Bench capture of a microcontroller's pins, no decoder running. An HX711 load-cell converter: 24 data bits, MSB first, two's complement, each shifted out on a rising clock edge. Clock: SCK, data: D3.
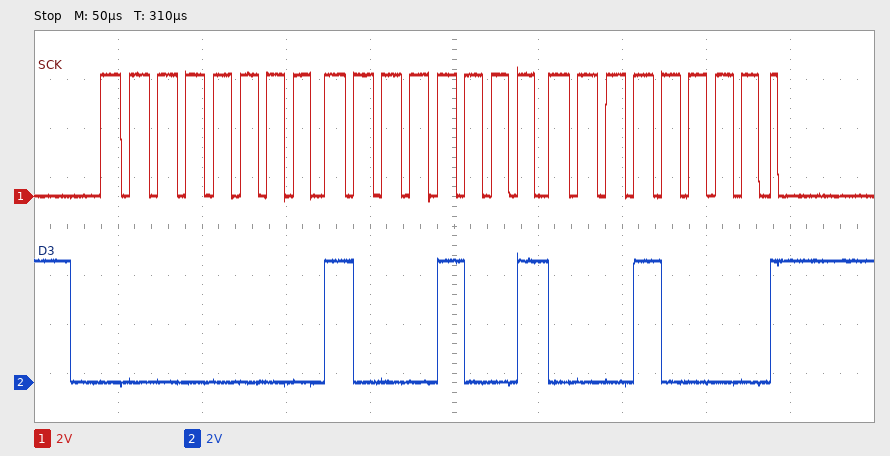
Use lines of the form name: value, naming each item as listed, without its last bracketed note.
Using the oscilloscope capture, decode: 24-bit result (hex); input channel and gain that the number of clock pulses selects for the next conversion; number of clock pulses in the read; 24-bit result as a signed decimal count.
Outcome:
24-bit result: 0x008910
input channel and gain that the number of clock pulses selects for the next conversion: channel A, gain 128
number of clock pulses in the read: 25
24-bit result as a signed decimal count: 35088
